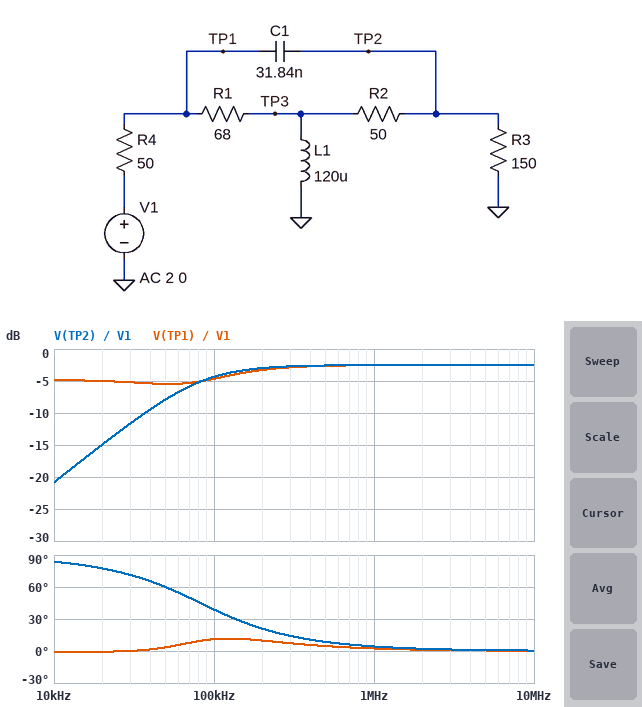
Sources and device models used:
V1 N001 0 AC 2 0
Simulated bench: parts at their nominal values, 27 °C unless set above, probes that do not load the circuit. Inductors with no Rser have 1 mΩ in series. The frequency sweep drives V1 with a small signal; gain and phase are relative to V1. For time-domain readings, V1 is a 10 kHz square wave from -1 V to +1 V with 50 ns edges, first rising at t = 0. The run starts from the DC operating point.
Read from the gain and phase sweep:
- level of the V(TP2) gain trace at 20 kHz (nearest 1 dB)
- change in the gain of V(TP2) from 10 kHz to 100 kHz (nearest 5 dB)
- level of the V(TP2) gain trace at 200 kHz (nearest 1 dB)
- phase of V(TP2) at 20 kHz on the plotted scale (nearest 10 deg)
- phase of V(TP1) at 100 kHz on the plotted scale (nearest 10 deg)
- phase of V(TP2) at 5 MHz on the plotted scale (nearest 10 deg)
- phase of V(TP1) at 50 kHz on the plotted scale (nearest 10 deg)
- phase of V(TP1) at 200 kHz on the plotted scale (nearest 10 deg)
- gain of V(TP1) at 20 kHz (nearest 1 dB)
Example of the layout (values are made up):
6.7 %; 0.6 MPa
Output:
-15 dB; 15 dB; -3 dB; 80 deg; 10 deg; 0 deg; 0 deg; 10 deg; -5 dB
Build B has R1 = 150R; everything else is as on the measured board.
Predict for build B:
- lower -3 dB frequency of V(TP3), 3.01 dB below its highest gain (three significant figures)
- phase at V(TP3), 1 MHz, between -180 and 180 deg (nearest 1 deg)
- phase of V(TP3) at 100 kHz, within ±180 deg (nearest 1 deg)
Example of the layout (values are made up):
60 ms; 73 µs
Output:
104 kHz; 7 deg; 59 deg
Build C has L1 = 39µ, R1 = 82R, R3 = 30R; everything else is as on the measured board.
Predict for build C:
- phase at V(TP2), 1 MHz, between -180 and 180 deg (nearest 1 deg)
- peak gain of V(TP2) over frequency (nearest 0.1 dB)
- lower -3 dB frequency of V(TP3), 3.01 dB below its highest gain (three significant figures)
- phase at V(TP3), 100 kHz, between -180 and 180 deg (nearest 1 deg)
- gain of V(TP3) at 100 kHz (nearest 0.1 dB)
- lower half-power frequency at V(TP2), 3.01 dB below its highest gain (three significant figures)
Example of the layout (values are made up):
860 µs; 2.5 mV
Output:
8 deg; -8.5 dB; 203 kHz; 64 deg; -15.6 dB; 138 kHz
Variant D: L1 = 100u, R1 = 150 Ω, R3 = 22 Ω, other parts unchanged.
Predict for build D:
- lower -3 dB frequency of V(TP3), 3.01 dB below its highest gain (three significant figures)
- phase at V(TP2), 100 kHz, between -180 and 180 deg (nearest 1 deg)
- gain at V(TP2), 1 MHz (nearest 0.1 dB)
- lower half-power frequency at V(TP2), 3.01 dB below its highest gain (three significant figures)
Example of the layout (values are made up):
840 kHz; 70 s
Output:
96.6 kHz; 43 deg; -10.3 dB; 93.7 kHz
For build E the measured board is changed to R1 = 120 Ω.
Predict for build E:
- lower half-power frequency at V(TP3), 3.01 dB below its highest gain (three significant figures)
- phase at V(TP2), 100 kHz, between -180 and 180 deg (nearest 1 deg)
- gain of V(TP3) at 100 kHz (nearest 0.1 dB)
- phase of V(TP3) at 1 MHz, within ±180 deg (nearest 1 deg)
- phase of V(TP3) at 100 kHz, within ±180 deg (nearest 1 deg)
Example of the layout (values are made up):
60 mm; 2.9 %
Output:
103 kHz; 40 deg; -5.7 dB; 6 deg; 56 deg
